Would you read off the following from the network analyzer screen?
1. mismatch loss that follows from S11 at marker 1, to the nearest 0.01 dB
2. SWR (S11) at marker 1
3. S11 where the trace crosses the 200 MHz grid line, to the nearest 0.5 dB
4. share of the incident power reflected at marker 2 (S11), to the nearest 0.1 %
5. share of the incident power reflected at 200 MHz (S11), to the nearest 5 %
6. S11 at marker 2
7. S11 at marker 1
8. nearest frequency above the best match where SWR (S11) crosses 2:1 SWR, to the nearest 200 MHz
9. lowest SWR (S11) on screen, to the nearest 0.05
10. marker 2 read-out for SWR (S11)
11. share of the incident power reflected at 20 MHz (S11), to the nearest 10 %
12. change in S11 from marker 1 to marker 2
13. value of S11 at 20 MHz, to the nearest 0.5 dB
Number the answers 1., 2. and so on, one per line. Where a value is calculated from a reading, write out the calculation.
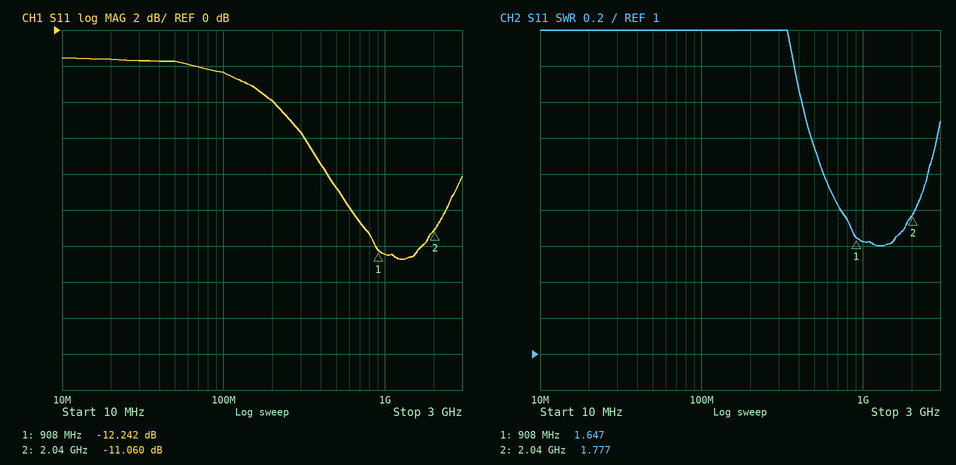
1. −10 log10(1 − 10^(-12.242/10)) ≈ 0.27 dB
2. 1.647
3. -4.0 dB
4. 10^(-11.06/10) ≈ 7.8 %
5. 10^(-4/10) ≈ 40 %
6. -11.060 dB
7. -12.242 dB
8. 2.6 GHz
9. 1.60
10. 1.777
11. 10^(-1.5/10) ≈ 70.8 %, so 70 % to the nearest 10 %
12. -11.06 − (-12.242) = 1.182 dB
13. -1.5 dB
